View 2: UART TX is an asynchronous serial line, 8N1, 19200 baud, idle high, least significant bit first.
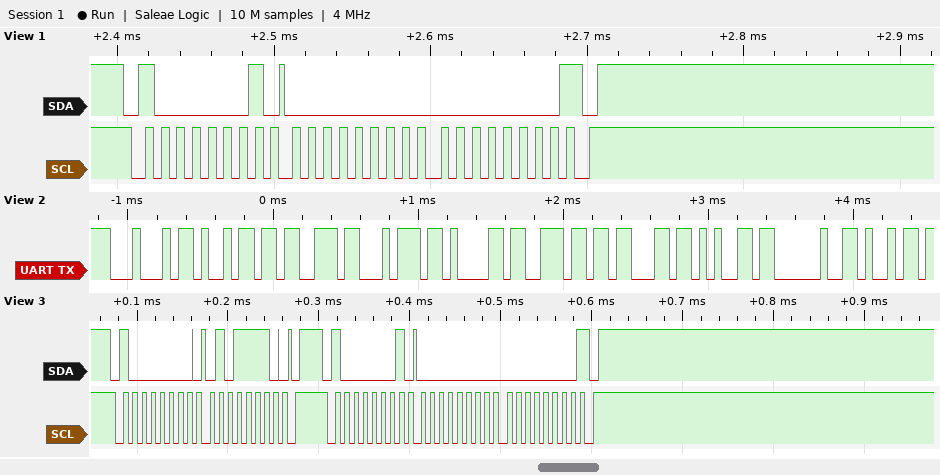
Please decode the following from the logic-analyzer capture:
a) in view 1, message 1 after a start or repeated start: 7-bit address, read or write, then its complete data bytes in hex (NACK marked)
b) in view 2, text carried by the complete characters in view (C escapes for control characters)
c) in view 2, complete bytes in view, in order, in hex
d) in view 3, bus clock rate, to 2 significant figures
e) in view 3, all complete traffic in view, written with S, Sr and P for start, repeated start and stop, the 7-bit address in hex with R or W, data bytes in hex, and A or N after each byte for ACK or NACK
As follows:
0x40 read: 00 00 NACK
"Distance i"
44 69 73 74 61 6E 63 65 20 69
100 kHz
S 40W A 5E A P S 40R A 00 A 00 N P
